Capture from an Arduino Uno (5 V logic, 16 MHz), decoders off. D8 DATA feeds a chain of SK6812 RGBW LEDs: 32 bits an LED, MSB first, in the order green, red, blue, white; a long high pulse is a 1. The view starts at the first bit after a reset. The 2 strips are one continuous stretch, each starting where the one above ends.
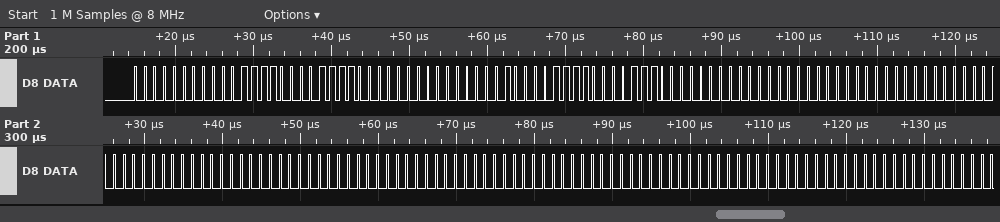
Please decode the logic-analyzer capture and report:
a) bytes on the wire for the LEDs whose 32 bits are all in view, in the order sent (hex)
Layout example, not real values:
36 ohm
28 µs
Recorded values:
00 1E 1E 00 02 1E 1C 00 00 00 00 00 00 00 00 00 00 00 00 00
